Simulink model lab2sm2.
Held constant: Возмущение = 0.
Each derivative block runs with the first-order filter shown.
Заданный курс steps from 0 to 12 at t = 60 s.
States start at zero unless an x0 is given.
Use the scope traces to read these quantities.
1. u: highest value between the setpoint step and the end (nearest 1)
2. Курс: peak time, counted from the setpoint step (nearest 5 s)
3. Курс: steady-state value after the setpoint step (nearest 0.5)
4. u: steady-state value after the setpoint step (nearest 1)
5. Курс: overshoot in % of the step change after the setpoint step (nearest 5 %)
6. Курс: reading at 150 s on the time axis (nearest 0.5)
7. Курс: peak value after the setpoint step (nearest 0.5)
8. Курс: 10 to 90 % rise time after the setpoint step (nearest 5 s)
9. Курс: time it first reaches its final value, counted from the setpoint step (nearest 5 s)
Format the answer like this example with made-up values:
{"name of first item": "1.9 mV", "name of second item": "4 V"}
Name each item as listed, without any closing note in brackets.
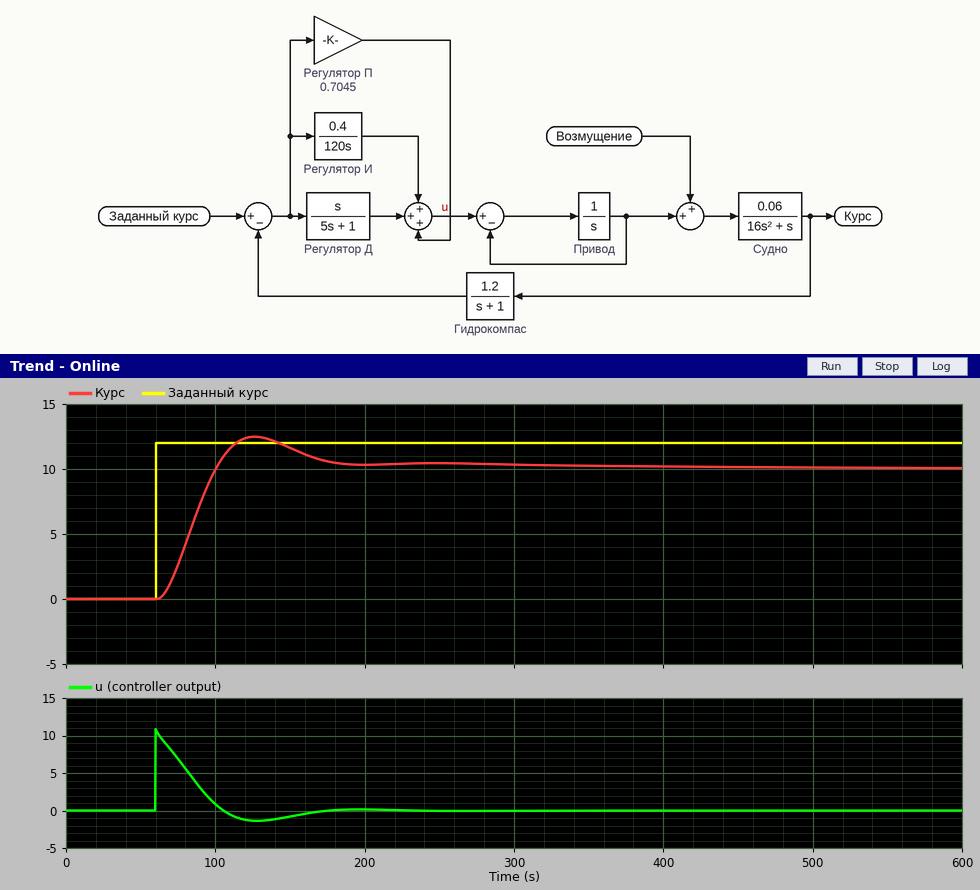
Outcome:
{"u: highest value between the setpoint step and the end": "11", "Курс: peak time, counted from the setpoint step": "65 s", "Курс: steady-state value after the setpoint step": "10.0", "u: steady-state value after the setpoint step": "0", "Курс: overshoot in % of the step change after the setpoint step": "25 %", "Курс: reading at 150 s on the time axis": "11.5", "Курс: peak value after the setpoint step": "12.5", "Курс: 10 to 90 % rise time after the setpoint step": "25 s", "Курс: time it first reaches its final value, counted from the setpoint step": "40 s"}
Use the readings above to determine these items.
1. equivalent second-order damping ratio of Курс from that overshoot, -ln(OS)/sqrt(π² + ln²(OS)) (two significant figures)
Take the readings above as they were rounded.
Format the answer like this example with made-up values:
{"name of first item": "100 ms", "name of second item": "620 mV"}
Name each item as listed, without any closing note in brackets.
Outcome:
{"equivalent second-order damping ratio of Курс from that overshoot, -ln(OS)/sqrt(π² + ln²(OS))": "0.40"}
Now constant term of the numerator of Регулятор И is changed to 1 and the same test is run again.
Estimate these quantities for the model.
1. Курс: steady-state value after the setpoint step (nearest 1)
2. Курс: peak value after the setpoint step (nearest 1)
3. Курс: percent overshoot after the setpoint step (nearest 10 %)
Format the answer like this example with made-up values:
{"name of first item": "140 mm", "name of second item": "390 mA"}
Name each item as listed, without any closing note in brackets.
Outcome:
{"Курс: steady-state value after the setpoint step": "10", "Курс: peak value after the setpoint step": "14", "Курс: percent overshoot after the setpoint step": "40 %"}
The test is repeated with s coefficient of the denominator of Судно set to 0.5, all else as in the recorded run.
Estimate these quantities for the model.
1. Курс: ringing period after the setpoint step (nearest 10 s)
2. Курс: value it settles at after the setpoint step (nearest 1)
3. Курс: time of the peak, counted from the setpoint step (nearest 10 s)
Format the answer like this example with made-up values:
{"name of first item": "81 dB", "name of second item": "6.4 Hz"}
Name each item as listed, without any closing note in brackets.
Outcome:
{"Курс: ringing period after the setpoint step": "120 s", "Курс: value it settles at after the setpoint step": "10", "Курс: time of the peak, counted from the setpoint step": "60 s"}
